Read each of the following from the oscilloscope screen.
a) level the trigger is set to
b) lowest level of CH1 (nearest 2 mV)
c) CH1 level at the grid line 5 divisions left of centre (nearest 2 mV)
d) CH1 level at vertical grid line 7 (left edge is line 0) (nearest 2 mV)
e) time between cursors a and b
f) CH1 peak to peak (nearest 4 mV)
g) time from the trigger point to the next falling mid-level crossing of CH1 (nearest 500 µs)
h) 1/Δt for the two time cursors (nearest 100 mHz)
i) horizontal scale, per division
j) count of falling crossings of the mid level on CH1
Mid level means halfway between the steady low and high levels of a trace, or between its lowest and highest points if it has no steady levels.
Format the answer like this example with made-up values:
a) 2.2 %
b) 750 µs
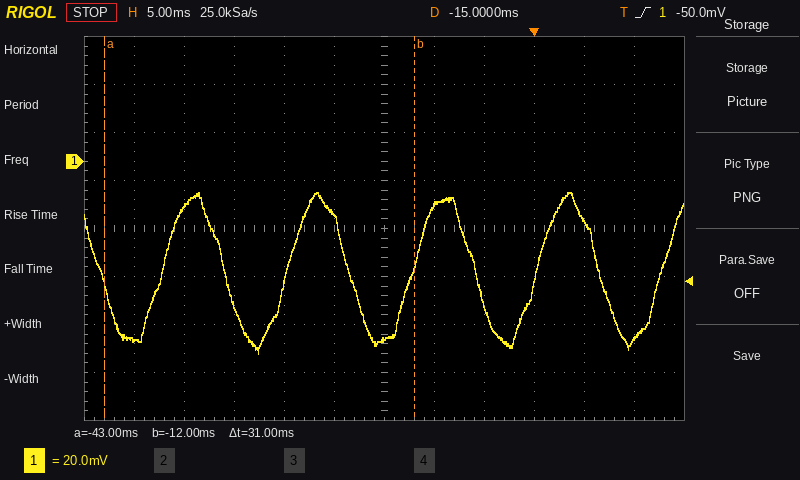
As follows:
a) -50.0 mV
b) -80 mV
c) -74 mV
d) -18 mV
e) 31 ms
f) 68 mV
g) 6.5 ms
h) 32.3 Hz
i) 5 ms
j) 5
